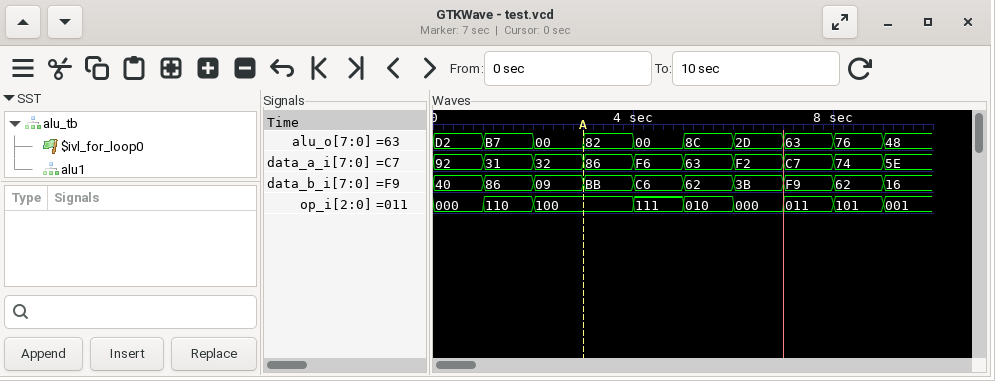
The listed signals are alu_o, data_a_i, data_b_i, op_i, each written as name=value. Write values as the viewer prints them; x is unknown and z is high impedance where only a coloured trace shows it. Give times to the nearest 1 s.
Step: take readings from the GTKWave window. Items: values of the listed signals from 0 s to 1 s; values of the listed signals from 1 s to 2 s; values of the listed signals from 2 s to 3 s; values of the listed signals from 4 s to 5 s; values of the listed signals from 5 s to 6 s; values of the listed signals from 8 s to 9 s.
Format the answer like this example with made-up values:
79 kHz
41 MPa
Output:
alu_o=D2, data_a_i=92, data_b_i=40, op_i=000
alu_o=B7, data_a_i=31, data_b_i=86, op_i=110
alu_o=00, data_a_i=32, data_b_i=09, op_i=100
alu_o=00, data_a_i=F6, data_b_i=C6, op_i=111
alu_o=8C, data_a_i=63, data_b_i=62, op_i=010
alu_o=76, data_a_i=74, data_b_i=62, op_i=101
